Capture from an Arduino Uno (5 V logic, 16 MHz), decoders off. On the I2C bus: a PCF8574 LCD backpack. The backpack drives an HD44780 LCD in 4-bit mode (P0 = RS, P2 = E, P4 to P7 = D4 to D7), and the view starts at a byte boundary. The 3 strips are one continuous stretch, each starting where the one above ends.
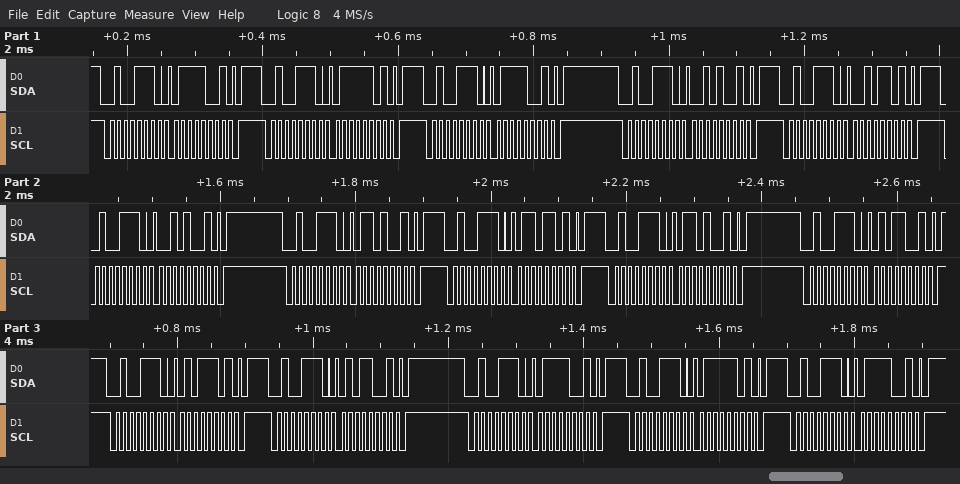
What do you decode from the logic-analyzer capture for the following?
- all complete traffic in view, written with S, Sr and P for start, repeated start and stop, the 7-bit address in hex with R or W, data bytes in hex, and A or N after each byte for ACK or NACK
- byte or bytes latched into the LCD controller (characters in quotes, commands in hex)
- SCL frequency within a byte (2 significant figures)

S 27W A 79 A P S 27W A 7D A P S 27W A 79 A P S 27W A 29 A P S 27W A 2D A P S 27W A 29 A P S 27W A 69 A P S 27W A 6D A P S 27W A 69 A P S 27W A 59 A P S 27W A 5D A P S 27W A 59 A P S 27W A 79 A P S 27W A 7D A P S 27W A 79 A P
'r' 'e'
100 kHz
